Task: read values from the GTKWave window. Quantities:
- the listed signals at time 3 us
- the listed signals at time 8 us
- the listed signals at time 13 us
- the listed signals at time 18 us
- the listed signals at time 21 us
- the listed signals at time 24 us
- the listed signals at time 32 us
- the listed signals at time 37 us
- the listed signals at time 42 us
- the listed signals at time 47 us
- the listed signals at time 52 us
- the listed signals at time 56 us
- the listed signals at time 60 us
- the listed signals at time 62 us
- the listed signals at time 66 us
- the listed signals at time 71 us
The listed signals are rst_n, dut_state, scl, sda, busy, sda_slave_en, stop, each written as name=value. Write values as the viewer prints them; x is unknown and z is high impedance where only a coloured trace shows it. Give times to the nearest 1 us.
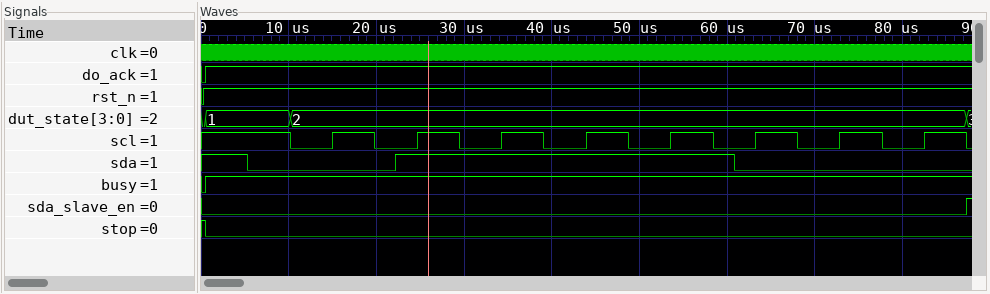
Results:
rst_n=1, dut_state=1, scl=1, sda=1, busy=1, sda_slave_en=0, stop=0
rst_n=1, dut_state=1, scl=1, sda=0, busy=1, sda_slave_en=0, stop=0
rst_n=1, dut_state=2, scl=0, sda=0, busy=1, sda_slave_en=0, stop=0
rst_n=1, dut_state=2, scl=1, sda=0, busy=1, sda_slave_en=0, stop=0
rst_n=1, dut_state=2, scl=0, sda=0, busy=1, sda_slave_en=0, stop=0
rst_n=1, dut_state=2, scl=0, sda=1, busy=1, sda_slave_en=0, stop=0
rst_n=1, dut_state=2, scl=0, sda=1, busy=1, sda_slave_en=0, stop=0
rst_n=1, dut_state=2, scl=1, sda=1, busy=1, sda_slave_en=0, stop=0
rst_n=1, dut_state=2, scl=0, sda=1, busy=1, sda_slave_en=0, stop=0
rst_n=1, dut_state=2, scl=1, sda=1, busy=1, sda_slave_en=0, stop=0
rst_n=1, dut_state=2, scl=0, sda=1, busy=1, sda_slave_en=0, stop=0
rst_n=1, dut_state=2, scl=1, sda=1, busy=1, sda_slave_en=0, stop=0
rst_n=1, dut_state=2, scl=0, sda=1, busy=1, sda_slave_en=0, stop=0
rst_n=1, dut_state=2, scl=0, sda=0, busy=1, sda_slave_en=0, stop=0
rst_n=1, dut_state=2, scl=1, sda=0, busy=1, sda_slave_en=0, stop=0
rst_n=1, dut_state=2, scl=0, sda=0, busy=1, sda_slave_en=0, stop=0
